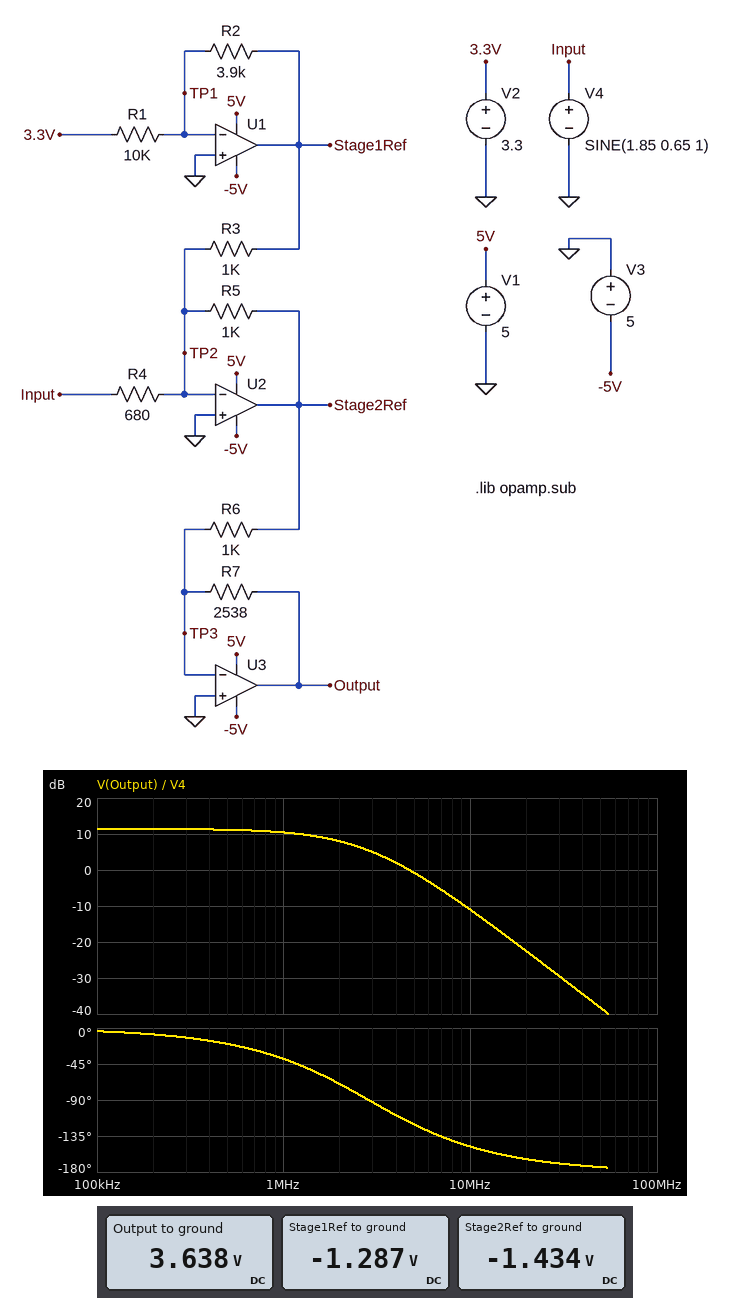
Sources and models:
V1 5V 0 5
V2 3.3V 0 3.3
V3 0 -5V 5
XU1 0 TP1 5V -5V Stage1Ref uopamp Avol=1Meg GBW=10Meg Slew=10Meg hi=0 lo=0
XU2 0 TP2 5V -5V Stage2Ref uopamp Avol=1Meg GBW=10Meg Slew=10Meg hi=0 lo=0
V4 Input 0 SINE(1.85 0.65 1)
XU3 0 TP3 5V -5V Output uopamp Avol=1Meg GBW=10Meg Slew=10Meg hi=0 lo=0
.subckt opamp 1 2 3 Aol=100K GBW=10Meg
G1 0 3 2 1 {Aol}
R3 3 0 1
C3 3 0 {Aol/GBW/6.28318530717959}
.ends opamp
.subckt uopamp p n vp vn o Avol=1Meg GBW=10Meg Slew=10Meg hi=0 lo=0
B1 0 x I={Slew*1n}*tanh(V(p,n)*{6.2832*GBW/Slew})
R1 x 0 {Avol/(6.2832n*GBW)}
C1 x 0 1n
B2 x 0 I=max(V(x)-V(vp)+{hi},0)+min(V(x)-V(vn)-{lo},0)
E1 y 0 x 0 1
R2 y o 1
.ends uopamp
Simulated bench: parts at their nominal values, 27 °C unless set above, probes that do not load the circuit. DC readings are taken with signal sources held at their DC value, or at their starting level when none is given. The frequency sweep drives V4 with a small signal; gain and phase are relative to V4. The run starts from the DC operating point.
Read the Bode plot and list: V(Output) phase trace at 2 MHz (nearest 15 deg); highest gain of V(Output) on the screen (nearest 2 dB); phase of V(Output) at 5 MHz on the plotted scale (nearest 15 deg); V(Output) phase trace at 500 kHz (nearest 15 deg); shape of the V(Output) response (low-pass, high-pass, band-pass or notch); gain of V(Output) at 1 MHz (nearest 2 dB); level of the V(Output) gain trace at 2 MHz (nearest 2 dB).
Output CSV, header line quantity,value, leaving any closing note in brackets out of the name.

quantity,value
V(Output) phase trace at 2 MHz,-75 deg
highest gain of V(Output) on the screen,12 dB
phase of V(Output) at 5 MHz on the plotted scale,-120 deg
V(Output) phase trace at 500 kHz,-15 deg
shape of the V(Output) response,low-pass
gain of V(Output) at 1 MHz,10 dB
level of the V(Output) gain trace at 2 MHz,8 dB
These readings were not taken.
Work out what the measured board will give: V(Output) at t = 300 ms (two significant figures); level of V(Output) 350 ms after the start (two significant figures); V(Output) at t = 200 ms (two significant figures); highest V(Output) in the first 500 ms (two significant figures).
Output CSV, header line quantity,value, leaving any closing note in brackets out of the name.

quantity,value
V(Output) at t = 300 ms,5.0 V
level of V(Output) 350 ms after the start,5.0 V
V(Output) at t = 200 ms,5.0 V
highest V(Output) in the first 500 ms,5.0 V
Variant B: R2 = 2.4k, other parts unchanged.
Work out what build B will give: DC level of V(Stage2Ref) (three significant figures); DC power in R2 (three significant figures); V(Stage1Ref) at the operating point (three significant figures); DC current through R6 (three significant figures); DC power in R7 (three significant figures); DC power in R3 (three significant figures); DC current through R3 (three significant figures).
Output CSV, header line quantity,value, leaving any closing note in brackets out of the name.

quantity,value
DC level of V(Stage2Ref),-1.93 V
DC power in R2,261 µW
V(Stage1Ref) at the operating point,-792 mV
DC current through R6,1.93 mA
DC power in R7,9.44 mW
DC power in R3,627 µW
DC current through R3,792 µA
